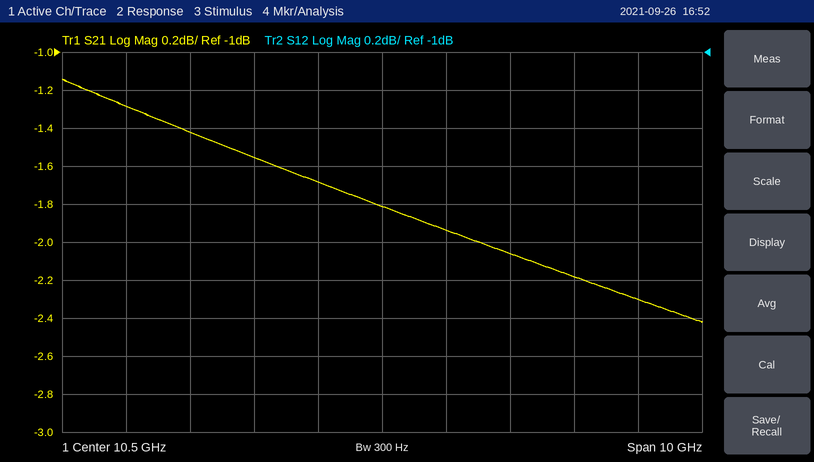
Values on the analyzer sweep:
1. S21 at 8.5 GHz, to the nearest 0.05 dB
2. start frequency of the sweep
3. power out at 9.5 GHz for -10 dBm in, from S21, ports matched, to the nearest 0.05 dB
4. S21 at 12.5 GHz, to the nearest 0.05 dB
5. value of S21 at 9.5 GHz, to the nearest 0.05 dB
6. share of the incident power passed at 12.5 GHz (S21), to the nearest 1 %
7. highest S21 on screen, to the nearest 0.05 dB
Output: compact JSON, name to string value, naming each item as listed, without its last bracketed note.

{"S21 at 8.5 GHz, to the nearest 0.05 dB": "-1.55 dB", "start frequency of the sweep": "5.5 GHz", "power out at 9.5 GHz for -10 dBm in, from S21, ports matched, to the nearest 0.05 dB": "-11.70 dBm", "S21 at 12.5 GHz, to the nearest 0.05 dB": "-2.05 dB", "value of S21 at 9.5 GHz, to the nearest 0.05 dB": "-1.70 dB", "share of the incident power passed at 12.5 GHz (S21), to the nearest 1 %": "62 %", "highest S21 on screen, to the nearest 0.05 dB": "-1.15 dB"}
